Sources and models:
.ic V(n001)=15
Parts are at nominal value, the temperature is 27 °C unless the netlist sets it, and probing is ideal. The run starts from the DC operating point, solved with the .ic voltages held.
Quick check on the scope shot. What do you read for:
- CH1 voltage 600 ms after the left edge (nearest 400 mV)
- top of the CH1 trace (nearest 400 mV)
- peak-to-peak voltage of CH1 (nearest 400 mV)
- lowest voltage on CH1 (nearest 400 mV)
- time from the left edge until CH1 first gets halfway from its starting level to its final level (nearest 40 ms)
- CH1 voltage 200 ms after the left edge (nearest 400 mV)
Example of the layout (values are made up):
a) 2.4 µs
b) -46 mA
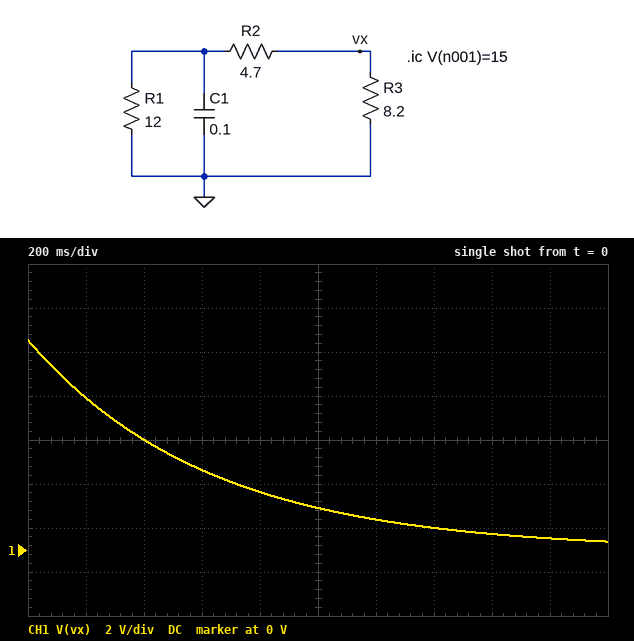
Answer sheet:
a) 3.6 V
b) 9.6 V
c) 9.2 V
d) 400 mV
e) 400 ms
f) 6.8 V
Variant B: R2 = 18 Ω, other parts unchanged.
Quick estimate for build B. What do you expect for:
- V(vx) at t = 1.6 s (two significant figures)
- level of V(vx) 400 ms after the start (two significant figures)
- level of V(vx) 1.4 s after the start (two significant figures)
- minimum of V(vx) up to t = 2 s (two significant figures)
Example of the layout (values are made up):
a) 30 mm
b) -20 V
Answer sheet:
a) 670 mV
b) 2.9 V
c) 860 mV
d) 410 mV
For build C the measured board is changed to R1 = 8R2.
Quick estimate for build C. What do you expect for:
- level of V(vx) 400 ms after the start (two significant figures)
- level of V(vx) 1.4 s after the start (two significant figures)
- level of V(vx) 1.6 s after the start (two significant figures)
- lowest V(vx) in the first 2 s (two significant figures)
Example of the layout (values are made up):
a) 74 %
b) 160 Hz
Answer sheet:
a) 4.3 V
b) 580 mV
c) 390 mV
d) 180 mV
